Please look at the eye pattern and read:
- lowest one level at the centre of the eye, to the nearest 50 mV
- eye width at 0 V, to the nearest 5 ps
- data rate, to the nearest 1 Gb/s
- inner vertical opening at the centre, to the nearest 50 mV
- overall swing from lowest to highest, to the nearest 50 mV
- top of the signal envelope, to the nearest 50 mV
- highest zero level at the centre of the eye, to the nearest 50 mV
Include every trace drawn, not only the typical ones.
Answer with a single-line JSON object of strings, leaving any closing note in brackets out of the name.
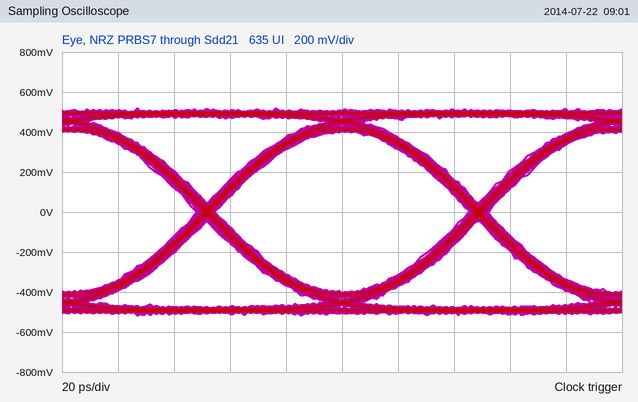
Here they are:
{"lowest one level at the centre of the eye, to the nearest 50 mV": "400 mV", "eye width at 0 V, to the nearest 5 ps": "90 ps", "data rate, to the nearest 1 Gb/s": "10 Gb/s", "inner vertical opening at the centre, to the nearest 50 mV": "800 mV", "overall swing from lowest to highest, to the nearest 50 mV": "1.05 V", "top of the signal envelope, to the nearest 50 mV": "500 mV", "highest zero level at the centre of the eye, to the nearest 50 mV": "-400 mV"}
